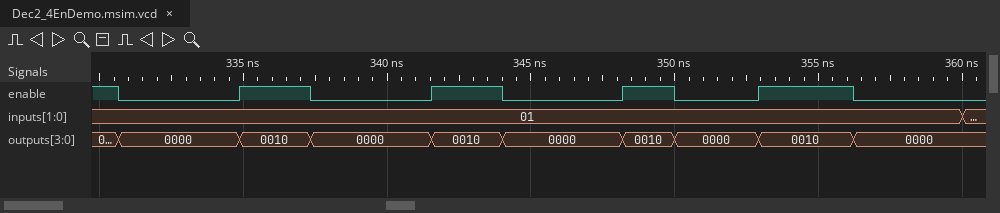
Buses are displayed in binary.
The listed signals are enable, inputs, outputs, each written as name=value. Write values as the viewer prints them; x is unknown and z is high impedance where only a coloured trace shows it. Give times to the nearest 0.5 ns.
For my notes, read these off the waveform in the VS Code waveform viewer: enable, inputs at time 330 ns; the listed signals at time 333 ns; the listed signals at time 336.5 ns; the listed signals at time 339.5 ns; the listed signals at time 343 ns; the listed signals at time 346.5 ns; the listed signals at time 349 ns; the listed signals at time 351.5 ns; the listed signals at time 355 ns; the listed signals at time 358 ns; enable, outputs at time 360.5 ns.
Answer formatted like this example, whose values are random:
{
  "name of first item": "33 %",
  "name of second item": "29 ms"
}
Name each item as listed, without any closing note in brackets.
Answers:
{
  "enable, inputs at time 330 ns": "enable=1, inputs=01",
  "the listed signals at time 333 ns": "enable=0, inputs=01, outputs=0000",
  "the listed signals at time 336.5 ns": "enable=1, inputs=01, outputs=0010",
  "the listed signals at time 339.5 ns": "enable=0, inputs=01, outputs=0000",
  "the listed signals at time 343 ns": "enable=1, inputs=01, outputs=0010",
  "the listed signals at time 346.5 ns": "enable=0, inputs=01, outputs=0000",
  "the listed signals at time 349 ns": "enable=1, inputs=01, outputs=0010",
  "the listed signals at time 351.5 ns": "enable=0, inputs=01, outputs=0000",
  "the listed signals at time 355 ns": "enable=1, inputs=01, outputs=0010",
  "the listed signals at time 358 ns": "enable=0, inputs=01, outputs=0000",
  "enable, outputs at time 360.5 ns": "enable=0, outputs=0000"
}
